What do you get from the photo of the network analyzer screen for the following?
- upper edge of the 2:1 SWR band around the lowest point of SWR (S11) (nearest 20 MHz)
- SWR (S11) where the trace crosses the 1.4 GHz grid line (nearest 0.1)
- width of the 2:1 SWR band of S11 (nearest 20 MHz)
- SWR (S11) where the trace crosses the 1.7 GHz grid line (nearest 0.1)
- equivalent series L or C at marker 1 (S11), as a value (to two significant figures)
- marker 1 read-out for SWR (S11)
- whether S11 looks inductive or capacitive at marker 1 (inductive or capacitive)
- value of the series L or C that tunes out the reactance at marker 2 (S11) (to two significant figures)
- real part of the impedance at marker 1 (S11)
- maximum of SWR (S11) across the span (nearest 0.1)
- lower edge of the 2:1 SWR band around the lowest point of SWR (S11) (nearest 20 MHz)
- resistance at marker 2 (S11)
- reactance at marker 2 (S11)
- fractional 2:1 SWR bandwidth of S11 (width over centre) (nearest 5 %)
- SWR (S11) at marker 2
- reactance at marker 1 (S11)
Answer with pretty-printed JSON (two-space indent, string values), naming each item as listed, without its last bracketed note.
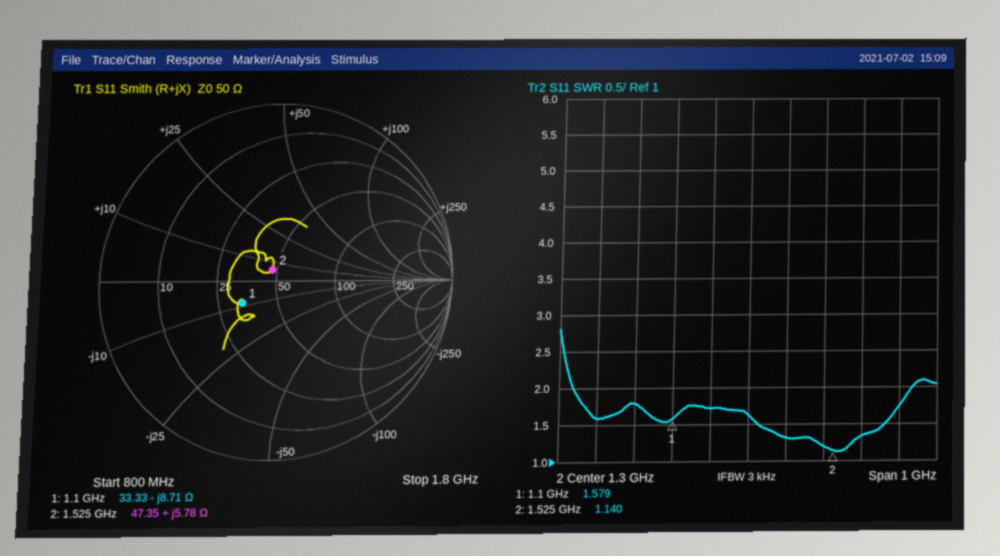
{
  "upper edge of the 2:1 SWR band around the lowest point of SWR (S11)": "1.74 GHz",
  "SWR (S11) where the trace crosses the 1.4 GHz grid line": "1.3",
  "width of the 2:1 SWR band of S11": "900 MHz",
  "SWR (S11) where the trace crosses the 1.7 GHz grid line": "1.7",
  "equivalent series L or C at marker 1 (S11), as a value": "17 pF",
  "marker 1 read-out for SWR": "1.579",
  "whether S11 looks inductive or capacitive at marker 1": "capacitive",
  "value of the series L or C that tunes out the reactance at marker 2 (S11)": "18 pF",
  "real part of the impedance at marker 1": "33.33 Ω",
  "maximum of SWR (S11) across the span": "2.8",
  "lower edge of the 2:1 SWR band around the lowest point of SWR (S11)": "840 MHz",
  "resistance at marker 2": "47.35 Ω",
  "reactance at marker 2": "+5.78 Ω",
  "fractional 2:1 SWR bandwidth of S11 (width over centre)": "70 %",
  "SWR (S11) at marker 2": "1.140",
  "reactance at marker 1": "-8.71 Ω"
}
